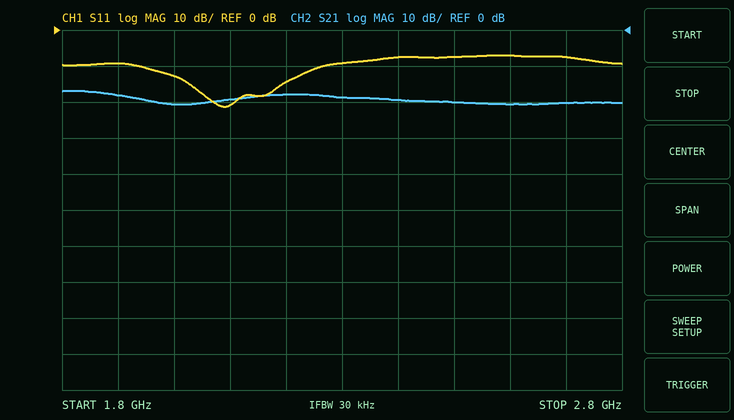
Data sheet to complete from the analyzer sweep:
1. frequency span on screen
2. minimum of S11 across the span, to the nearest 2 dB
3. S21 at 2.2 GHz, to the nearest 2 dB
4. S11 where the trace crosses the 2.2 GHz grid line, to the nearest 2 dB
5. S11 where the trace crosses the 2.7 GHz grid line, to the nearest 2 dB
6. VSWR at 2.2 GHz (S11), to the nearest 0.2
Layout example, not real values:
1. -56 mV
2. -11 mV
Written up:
1. 1 GHz
2. -22 dB
3. -18 dB
4. -14 dB
5. -8 dB
6. 1.4
